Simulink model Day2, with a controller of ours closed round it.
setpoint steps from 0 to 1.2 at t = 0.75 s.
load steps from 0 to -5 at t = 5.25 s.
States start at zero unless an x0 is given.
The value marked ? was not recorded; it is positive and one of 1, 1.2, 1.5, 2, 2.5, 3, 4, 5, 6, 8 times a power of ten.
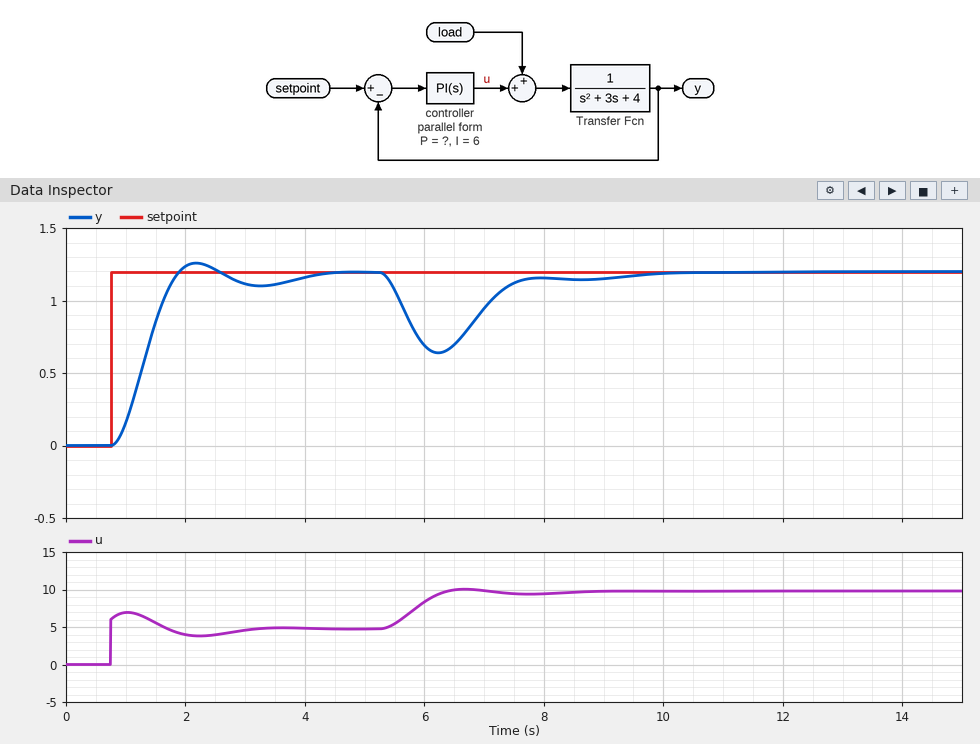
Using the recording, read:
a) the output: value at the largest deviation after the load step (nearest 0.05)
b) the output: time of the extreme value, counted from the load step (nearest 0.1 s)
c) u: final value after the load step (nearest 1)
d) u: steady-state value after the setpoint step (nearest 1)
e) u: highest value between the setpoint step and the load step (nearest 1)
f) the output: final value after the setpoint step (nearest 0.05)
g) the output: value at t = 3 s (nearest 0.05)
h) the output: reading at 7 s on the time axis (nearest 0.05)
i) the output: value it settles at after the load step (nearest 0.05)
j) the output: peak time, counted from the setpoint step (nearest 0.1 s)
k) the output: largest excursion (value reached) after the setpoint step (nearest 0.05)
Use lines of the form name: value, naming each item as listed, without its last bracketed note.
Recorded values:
the output: value at the largest deviation after the load step: 0.65
the output: time of the extreme value, counted from the load step: 1.0 s
u: final value after the load step: 10
u: steady-state value after the setpoint step: 5
u: highest value between the setpoint step and the load step: 7
the output: final value after the setpoint step: 1.20
the output: value at t = 3 s: 1.10
the output: reading at 7 s on the time axis: 0.95
the output: value it settles at after the load step: 1.20
the output: peak time, counted from the setpoint step: 1.4 s
the output: largest excursion (value reached) after the setpoint step: 1.25
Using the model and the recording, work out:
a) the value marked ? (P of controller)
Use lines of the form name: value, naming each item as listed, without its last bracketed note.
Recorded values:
the value marked ?: 5
